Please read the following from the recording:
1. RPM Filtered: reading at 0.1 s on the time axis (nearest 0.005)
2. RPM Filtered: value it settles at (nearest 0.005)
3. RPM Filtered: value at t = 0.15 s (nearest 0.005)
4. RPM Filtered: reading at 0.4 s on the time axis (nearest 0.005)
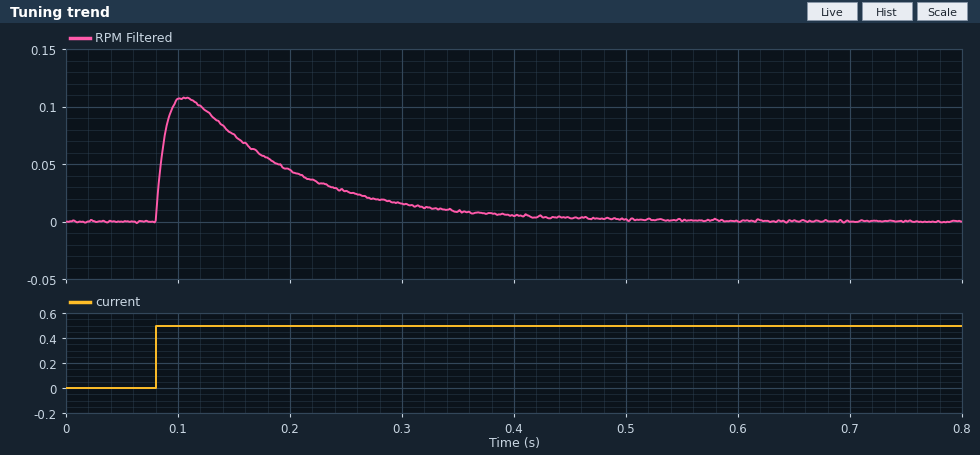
0.105
0.000
0.075
0.005
